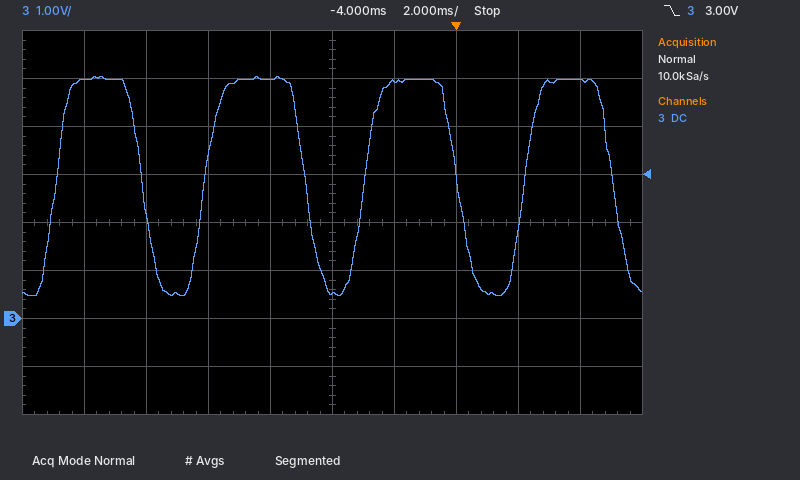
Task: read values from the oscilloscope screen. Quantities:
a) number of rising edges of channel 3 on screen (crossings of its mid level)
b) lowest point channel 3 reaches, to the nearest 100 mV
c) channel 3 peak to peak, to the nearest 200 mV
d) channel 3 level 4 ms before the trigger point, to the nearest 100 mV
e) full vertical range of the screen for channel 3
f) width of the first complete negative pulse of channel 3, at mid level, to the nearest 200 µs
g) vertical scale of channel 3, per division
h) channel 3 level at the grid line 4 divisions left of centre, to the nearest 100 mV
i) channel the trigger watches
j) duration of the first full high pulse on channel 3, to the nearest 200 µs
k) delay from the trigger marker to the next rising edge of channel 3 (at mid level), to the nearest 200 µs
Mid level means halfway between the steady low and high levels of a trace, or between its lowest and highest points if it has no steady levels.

4
500 mV
4.6 V
500 mV
8 V
2.0 ms
1 V
5.0 V
channel 3
2.8 ms
2.2 ms
